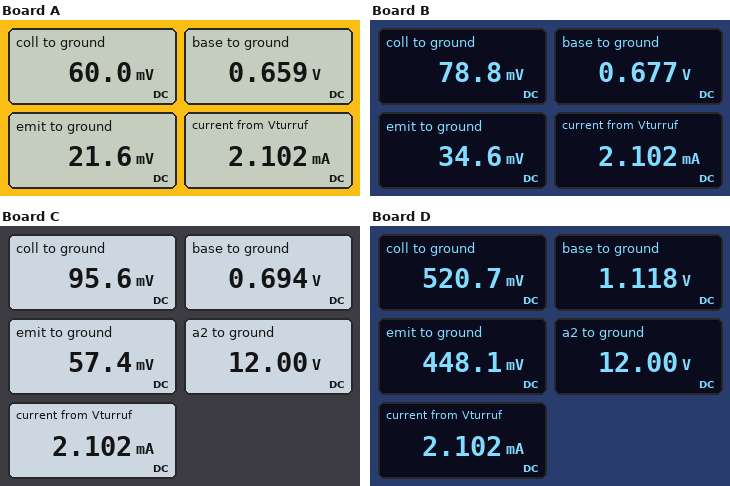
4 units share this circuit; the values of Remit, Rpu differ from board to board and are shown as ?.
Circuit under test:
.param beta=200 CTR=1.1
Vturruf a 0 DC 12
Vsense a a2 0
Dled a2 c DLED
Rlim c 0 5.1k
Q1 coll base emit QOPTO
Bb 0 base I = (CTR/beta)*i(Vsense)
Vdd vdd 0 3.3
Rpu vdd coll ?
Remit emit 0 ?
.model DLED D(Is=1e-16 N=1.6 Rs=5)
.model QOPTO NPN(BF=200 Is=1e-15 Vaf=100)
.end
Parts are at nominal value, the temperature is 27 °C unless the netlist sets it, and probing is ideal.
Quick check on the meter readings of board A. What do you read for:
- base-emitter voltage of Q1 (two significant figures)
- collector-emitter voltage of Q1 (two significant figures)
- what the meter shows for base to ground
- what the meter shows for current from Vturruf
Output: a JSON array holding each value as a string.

["640 mV", "38 mV", "0.659 V", "2.102 mA"]
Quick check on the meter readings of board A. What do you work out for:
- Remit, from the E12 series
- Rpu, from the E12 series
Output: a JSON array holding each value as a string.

["560 Ω", "120 kΩ"]
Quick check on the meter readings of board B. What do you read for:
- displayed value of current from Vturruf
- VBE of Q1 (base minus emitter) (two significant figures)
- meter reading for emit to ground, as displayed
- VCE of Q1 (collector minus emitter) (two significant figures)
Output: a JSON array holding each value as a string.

["2.102 mA", "640 mV", "34.6 mV", "44 mV"]
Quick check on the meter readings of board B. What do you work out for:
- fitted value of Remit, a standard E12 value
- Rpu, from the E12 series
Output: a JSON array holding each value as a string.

["680 Ω", "82 kΩ"]
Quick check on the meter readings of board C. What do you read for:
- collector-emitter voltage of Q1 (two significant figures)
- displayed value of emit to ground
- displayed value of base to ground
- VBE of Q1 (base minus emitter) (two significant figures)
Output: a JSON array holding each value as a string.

["38 mV", "57.4 mV", "0.694 V", "640 mV"]
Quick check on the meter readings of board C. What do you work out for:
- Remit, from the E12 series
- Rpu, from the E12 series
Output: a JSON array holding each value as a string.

["1.5 kΩ", "120 kΩ"]
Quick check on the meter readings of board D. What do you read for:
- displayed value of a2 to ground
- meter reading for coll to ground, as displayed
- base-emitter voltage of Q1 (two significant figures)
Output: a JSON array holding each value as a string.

["12.00 V", "520.7 mV", "670 mV"]
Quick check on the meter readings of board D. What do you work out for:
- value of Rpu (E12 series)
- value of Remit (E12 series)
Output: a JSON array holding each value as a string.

["18 kΩ", "2.7 kΩ"]
